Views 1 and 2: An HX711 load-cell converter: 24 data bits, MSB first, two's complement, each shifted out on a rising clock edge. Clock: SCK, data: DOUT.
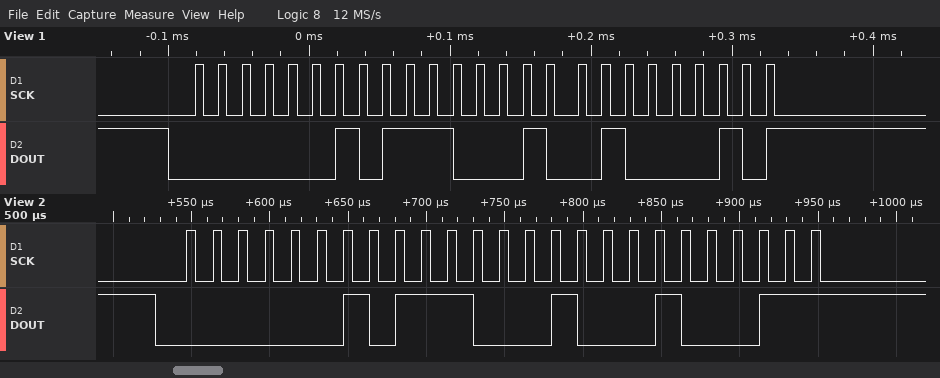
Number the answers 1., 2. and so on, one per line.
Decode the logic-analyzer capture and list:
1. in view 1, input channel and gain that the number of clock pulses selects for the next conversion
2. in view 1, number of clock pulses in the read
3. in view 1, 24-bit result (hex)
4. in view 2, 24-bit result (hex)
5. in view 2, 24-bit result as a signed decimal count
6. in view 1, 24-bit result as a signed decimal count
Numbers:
1. channel A, gain 128
2. 25
3. 0x02E242
4. 0x02E223
5. 188963
6. 188994
